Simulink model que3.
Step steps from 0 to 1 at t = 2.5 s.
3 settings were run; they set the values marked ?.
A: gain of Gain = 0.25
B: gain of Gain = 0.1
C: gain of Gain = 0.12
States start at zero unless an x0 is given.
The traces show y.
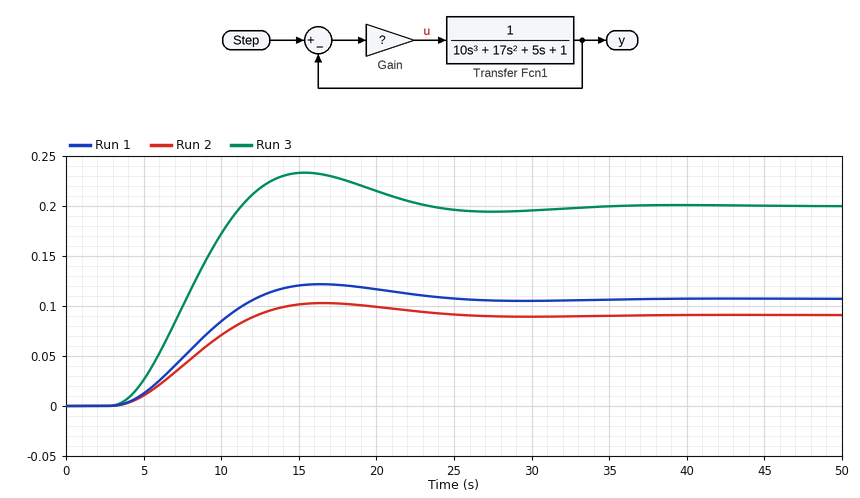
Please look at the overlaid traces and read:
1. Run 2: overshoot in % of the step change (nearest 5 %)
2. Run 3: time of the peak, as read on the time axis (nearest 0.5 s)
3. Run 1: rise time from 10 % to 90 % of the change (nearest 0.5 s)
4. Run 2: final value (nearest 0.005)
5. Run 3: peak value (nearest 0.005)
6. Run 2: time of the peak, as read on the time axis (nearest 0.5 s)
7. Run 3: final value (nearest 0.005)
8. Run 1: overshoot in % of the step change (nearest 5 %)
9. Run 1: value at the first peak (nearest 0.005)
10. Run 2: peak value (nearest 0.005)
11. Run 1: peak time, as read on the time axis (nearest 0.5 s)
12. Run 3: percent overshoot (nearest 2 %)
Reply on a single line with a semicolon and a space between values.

15 %; 15.5 s; 6.0 s; 0.090; 0.235; 16.5 s; 0.200; 15 %; 0.120; 0.105; 16.5 s; 16 %
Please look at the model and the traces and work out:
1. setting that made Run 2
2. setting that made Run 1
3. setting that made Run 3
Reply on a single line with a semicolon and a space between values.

B; C; A
